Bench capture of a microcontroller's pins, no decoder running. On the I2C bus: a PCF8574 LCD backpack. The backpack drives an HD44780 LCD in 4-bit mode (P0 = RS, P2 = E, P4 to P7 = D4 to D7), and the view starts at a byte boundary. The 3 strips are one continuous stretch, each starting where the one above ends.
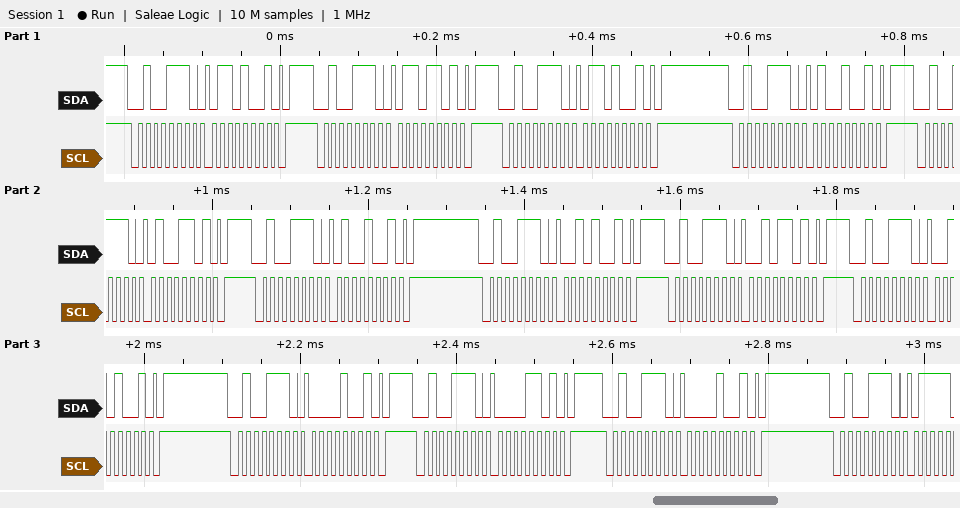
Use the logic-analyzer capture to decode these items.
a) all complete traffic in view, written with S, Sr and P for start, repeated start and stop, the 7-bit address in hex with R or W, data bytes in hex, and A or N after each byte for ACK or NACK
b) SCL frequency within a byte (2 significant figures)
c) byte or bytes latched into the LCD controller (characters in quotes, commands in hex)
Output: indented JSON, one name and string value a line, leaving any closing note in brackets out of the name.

{
  "all complete traffic in view, written with S, Sr and P for start, repeated start and stop, the 7-bit address in hex with R or W, data bytes in hex, and A or N after each byte for ACK or NACK": "S 27W A 69 A P S 27W A 6D A P S 27W A 69 A P S 27W A 49 A P S 27W A 4D A P S 27W A 49 A P S 27W A 29 A P S 27W A 2D A P S 27W A 29 A P S 27W A 09 A P S 27W A 0D A P S 27W A 09 A P S 27W A",
  "SCL frequency within a byte": "100 kHz",
  "byte or bytes latched into the LCD controller": "'d' ' '"
}
